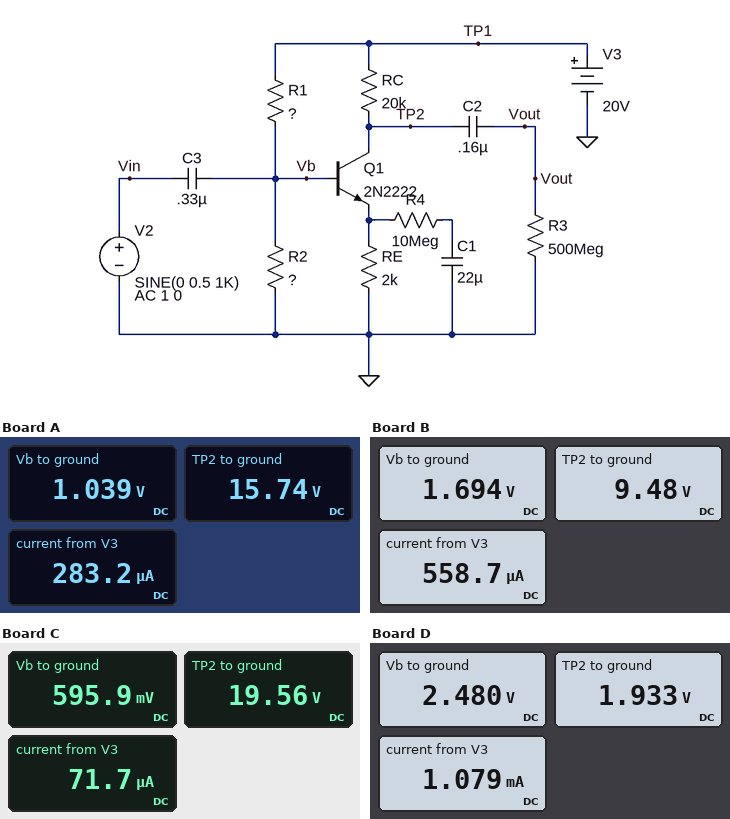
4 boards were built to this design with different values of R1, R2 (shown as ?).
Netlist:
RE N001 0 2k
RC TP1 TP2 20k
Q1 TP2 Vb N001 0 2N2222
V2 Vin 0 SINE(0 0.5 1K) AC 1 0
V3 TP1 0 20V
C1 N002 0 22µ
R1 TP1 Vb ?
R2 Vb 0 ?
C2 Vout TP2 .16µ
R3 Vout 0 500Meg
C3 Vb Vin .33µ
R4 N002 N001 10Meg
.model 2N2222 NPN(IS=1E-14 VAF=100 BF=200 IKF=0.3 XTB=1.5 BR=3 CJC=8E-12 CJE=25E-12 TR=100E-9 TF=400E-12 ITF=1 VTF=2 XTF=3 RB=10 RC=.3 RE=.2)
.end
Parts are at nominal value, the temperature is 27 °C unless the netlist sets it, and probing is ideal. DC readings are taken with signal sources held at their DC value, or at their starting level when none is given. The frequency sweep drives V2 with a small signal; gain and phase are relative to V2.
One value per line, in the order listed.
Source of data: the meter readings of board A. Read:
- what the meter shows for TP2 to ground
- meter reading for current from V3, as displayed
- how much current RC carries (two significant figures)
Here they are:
15.74 V
283.2 µA
210 µA
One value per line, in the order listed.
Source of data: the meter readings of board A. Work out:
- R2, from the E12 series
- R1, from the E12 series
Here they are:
15 kΩ
270 kΩ
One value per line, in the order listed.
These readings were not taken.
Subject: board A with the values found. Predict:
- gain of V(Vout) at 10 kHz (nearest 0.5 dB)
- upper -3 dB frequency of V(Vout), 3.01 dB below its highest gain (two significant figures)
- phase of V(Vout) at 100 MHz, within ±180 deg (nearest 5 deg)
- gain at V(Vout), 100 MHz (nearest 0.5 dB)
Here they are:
19.5 dB
2.7 MHz
5 deg
0.5 dB
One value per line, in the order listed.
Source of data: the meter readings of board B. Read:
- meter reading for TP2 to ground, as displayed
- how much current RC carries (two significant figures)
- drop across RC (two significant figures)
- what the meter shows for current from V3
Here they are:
9.48 V
530 µA
11 V
558.7 µA
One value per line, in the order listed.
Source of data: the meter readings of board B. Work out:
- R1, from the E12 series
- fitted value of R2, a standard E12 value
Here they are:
560 kΩ
56 kΩ
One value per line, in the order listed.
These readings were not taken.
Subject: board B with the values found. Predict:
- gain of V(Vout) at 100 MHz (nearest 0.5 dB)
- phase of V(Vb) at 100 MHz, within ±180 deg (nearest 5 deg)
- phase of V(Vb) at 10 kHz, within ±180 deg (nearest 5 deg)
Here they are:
1.0 dB
0 deg
0 deg
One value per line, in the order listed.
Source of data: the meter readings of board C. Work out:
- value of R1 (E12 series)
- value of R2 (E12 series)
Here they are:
390 kΩ
12 kΩ
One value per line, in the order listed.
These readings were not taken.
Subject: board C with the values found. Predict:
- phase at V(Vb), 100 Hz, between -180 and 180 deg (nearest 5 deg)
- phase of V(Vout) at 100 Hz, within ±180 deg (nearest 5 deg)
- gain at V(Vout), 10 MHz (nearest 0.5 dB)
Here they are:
25 deg
-155 deg
5.0 dB
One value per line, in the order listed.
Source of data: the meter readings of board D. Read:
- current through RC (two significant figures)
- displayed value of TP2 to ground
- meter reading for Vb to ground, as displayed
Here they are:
900 µA
1.933 V
2.480 V
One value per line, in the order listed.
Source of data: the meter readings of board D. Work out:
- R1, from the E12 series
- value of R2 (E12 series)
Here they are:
100 kΩ
15 kΩ
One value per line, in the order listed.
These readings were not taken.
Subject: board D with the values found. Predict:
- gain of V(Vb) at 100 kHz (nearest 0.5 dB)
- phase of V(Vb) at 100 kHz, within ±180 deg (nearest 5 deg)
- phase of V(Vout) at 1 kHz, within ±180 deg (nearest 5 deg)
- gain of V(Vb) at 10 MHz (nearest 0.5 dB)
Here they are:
0 dB
0 deg
-165 deg
0 dB
